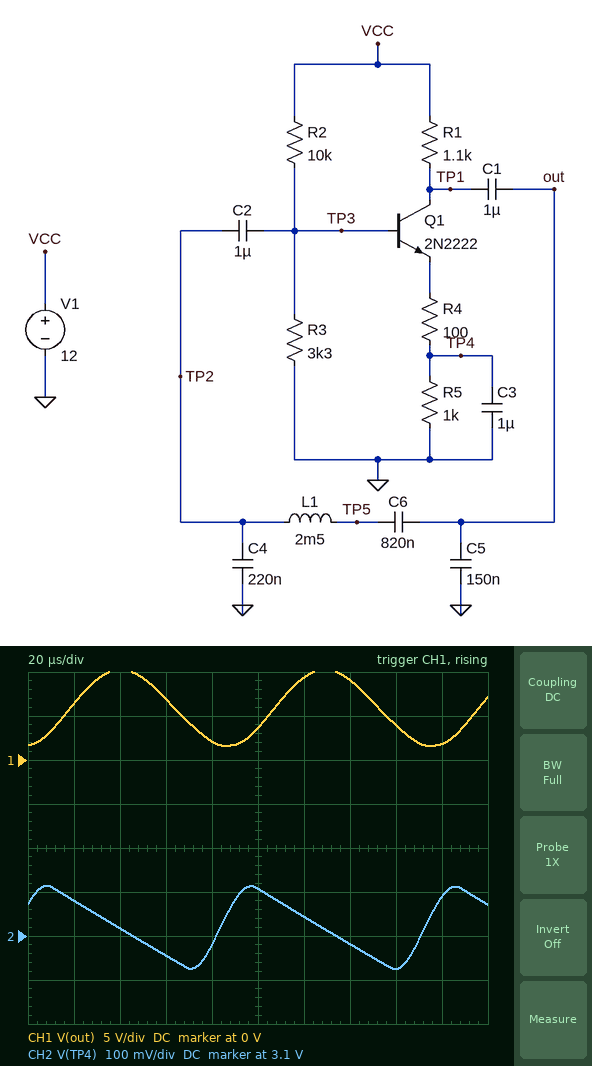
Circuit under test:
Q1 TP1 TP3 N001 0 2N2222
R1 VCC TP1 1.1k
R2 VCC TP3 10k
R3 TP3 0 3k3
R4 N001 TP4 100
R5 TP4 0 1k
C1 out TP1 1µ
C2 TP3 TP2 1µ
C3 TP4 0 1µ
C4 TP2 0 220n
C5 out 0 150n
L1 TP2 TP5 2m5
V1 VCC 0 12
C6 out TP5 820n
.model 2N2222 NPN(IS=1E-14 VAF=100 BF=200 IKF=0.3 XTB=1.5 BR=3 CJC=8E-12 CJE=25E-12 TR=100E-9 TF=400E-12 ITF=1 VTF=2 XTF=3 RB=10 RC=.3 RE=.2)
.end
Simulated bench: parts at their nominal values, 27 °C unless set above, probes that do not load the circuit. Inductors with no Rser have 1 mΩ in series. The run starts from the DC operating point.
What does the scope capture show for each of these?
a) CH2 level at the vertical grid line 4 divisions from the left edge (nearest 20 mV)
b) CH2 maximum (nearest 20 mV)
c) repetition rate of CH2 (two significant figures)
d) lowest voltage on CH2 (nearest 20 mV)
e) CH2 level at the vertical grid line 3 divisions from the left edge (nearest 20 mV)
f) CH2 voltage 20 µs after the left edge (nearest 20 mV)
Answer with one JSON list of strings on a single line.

["3.08 V", "3.22 V", "11 kHz", "3.02 V", "3.06 V", "3.18 V"]
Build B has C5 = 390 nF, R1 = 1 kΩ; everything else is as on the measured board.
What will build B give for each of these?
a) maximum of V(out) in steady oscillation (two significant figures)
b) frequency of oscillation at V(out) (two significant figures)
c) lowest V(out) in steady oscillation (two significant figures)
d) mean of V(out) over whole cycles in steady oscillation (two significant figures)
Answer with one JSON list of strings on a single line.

["7.4 V", "9.2 kHz", "2.4 V", "4.9 V"]
